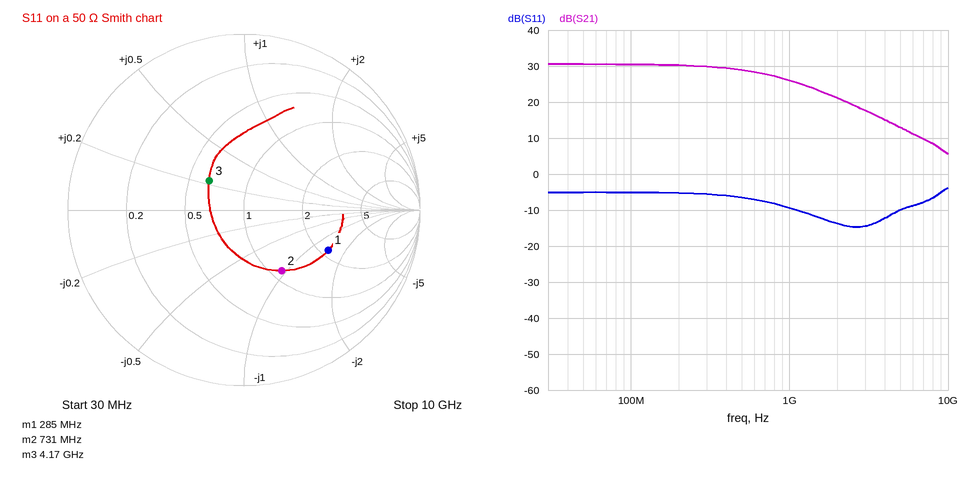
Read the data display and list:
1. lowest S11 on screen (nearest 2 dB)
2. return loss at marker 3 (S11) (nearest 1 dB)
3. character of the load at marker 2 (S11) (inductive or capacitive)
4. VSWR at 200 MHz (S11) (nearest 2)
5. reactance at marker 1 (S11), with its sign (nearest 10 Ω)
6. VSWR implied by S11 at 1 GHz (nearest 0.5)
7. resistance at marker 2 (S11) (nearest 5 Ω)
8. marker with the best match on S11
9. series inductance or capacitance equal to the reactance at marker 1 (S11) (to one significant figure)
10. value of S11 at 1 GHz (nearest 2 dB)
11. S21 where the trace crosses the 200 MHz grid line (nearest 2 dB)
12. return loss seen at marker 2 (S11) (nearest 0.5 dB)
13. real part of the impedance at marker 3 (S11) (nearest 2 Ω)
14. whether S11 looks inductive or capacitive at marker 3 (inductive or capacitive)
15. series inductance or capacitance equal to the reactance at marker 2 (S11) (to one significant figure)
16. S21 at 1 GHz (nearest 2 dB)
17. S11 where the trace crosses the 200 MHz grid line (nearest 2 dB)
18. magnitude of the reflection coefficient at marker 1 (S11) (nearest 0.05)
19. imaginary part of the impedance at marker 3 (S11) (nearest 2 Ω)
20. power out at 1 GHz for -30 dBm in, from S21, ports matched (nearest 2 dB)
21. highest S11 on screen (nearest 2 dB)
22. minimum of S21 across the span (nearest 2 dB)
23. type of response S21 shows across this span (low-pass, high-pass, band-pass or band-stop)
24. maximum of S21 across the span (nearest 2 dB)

-14 dB
12 dB
capacitive
4
-70 Ω
2.0
55 Ω
marker 3
8 pF
-10 dB
30 dB
8.0 dB
32 Ω
inductive
5 pF
26 dB
-6 dB
0.55
+12 Ω
-4 dBm
-4 dB
6 dB
low-pass
30 dB
